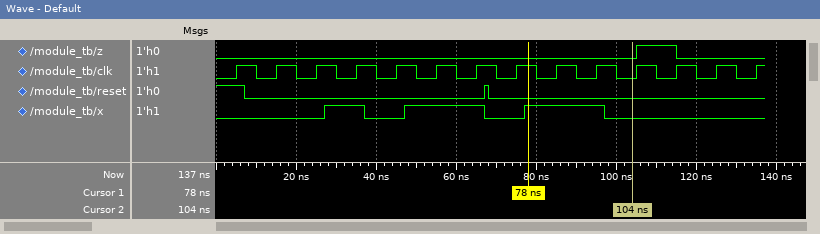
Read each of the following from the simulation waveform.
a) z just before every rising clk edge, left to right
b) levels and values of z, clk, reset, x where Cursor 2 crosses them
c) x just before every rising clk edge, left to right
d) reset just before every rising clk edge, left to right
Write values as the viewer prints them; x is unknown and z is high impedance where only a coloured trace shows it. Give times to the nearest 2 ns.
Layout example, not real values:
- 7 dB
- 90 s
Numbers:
- 0 0 0 0 0 0 0 0 0 0 0 1 0 0
- z=0, clk=0, reset=0, x=0
- 0 0 0 1 0 1 1 0 1 1 0 0 0 0
- 1 0 0 0 0 0 0 0 0 0 0 0 0 0
